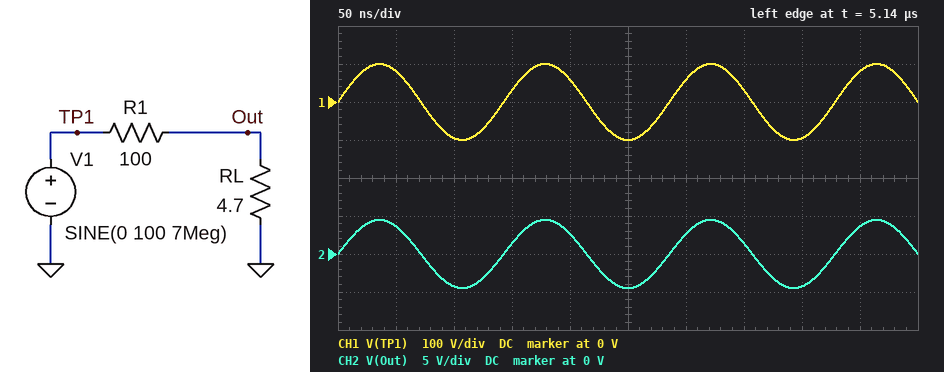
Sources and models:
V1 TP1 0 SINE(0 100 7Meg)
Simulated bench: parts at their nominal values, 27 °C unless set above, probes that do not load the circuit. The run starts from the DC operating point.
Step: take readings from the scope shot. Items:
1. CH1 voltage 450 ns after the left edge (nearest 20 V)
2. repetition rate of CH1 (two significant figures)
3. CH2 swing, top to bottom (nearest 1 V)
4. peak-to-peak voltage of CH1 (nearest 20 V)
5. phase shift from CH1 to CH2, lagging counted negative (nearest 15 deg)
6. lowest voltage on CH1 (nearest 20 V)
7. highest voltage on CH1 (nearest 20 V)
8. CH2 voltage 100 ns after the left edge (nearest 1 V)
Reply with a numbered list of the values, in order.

1. 80 V
2. 7.0 MHz
3. 9 V
4. 200 V
5. 0 deg
6. -100 V
7. 100 V
8. -4 V
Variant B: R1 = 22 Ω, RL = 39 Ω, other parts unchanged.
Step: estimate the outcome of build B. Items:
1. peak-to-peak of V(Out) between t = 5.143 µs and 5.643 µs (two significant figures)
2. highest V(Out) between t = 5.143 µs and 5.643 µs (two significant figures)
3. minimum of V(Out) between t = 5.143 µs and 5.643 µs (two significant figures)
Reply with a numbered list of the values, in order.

1. 130 V
2. 64 V
3. -64 V
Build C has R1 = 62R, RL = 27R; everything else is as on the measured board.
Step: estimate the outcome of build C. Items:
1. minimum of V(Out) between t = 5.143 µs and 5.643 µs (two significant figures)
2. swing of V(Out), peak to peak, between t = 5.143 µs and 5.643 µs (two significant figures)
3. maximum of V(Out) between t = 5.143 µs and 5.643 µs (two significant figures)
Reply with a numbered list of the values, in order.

1. -30 V
2. 61 V
3. 30 V
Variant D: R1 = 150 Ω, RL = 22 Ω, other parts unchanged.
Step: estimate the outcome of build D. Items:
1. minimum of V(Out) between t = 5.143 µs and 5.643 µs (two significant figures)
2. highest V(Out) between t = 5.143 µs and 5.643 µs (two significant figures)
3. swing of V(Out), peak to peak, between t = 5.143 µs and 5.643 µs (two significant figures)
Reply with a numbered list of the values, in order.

1. -13 V
2. 13 V
3. 26 V
